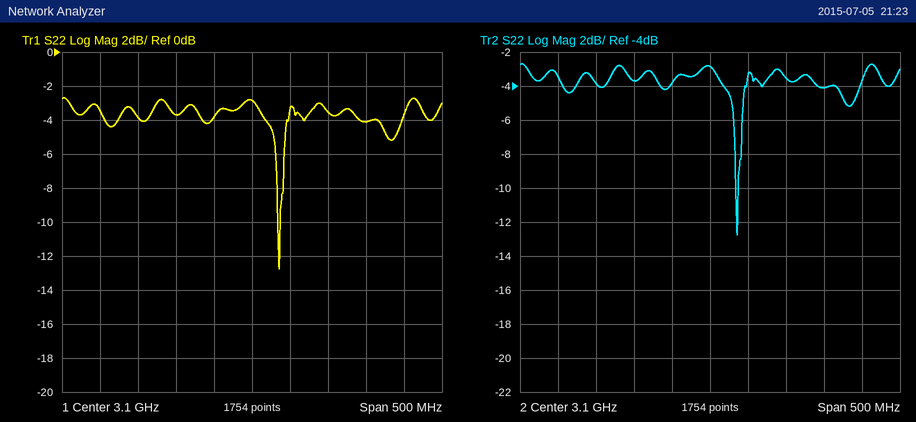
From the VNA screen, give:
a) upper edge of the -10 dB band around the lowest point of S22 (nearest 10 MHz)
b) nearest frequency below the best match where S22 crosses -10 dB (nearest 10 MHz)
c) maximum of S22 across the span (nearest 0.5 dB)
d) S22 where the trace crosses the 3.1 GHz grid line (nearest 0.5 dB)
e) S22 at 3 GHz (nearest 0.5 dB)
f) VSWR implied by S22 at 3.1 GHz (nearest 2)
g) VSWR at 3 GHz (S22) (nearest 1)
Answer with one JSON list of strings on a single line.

["3.14 GHz", "3.13 GHz", "-2.5 dB", "-3.0 dB", "-3.5 dB", "6", "5"]
